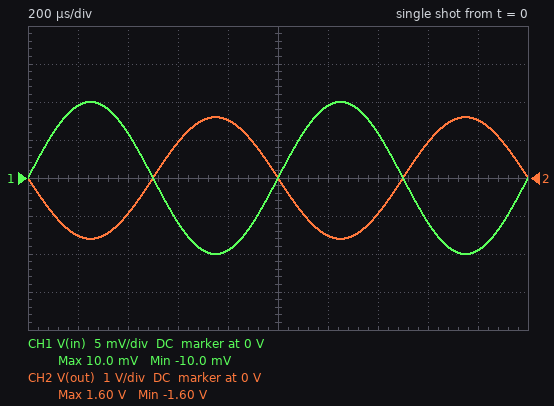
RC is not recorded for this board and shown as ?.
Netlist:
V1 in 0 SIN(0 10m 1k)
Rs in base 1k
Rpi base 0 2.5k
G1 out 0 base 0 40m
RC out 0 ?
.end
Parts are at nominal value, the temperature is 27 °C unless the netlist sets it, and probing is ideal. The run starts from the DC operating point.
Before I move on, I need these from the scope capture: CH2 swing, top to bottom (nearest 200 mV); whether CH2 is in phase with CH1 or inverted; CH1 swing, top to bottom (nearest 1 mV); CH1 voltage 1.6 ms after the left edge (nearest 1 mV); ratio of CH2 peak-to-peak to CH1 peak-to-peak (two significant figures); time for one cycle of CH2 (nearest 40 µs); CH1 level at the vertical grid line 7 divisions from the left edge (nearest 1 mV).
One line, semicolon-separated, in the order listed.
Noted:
3.2 V; inverted; 20 mV; -6 mV; 160; 1.00 ms; 6 mV
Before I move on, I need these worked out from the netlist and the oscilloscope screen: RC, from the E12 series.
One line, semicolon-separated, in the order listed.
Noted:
5.6 kΩ
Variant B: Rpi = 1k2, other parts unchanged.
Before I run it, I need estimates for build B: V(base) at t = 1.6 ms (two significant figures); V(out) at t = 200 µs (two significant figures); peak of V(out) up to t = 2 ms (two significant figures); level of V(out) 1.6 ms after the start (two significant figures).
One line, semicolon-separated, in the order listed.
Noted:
-3.2 mV; -1.2 V; 1.2 V; 720 mV
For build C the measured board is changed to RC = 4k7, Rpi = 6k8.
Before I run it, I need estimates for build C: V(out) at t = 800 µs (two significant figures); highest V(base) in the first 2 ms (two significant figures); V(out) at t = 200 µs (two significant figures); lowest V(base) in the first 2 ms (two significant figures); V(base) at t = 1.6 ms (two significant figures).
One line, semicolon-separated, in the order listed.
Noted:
1.6 V; 8.7 mV; -1.6 V; -8.7 mV; -5.1 mV
